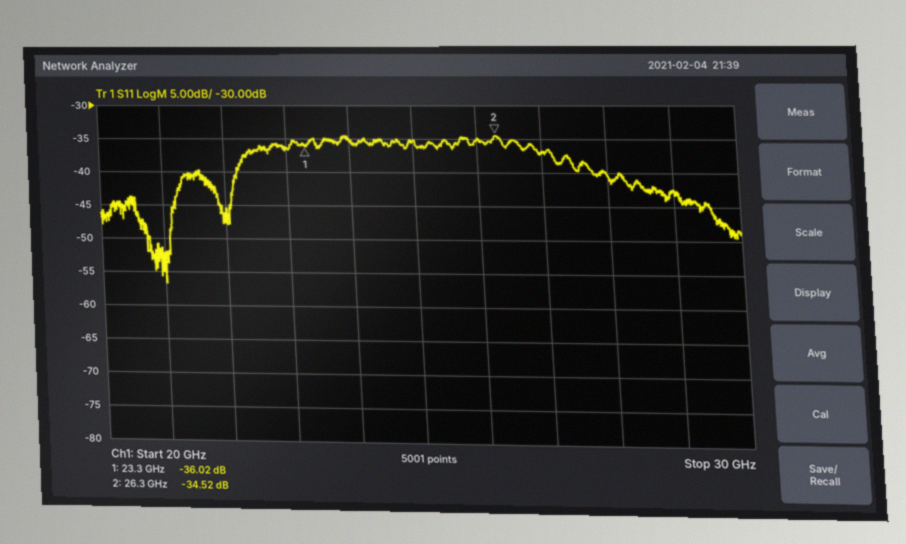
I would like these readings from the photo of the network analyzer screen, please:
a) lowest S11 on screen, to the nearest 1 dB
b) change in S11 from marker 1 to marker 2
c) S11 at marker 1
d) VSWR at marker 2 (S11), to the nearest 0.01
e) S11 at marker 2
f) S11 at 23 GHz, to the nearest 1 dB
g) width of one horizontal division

-57 dB
1.50 dB
-36.02 dB
1.04
-34.52 dB
-36 dB
1 GHz
